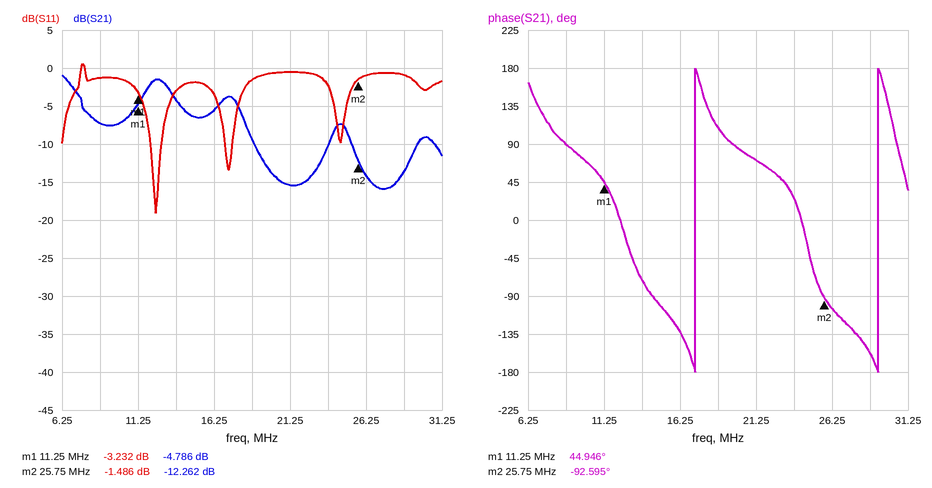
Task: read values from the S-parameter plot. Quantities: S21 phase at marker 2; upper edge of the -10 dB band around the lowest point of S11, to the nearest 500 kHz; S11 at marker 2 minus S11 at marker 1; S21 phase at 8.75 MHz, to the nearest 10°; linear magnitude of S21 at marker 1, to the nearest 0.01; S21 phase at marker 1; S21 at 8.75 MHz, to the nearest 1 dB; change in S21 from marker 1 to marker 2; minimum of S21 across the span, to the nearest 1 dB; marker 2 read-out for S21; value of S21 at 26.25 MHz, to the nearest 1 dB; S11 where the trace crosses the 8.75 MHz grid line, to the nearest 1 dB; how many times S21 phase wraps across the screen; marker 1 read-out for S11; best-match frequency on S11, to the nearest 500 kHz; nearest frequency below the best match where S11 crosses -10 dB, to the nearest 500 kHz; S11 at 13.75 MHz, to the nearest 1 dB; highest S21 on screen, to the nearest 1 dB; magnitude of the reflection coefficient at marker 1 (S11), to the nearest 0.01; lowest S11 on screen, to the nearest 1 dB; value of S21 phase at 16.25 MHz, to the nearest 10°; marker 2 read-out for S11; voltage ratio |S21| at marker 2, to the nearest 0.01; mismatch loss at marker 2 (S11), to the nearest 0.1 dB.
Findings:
-92.595°
13.0 MHz
1.746 dB
90°
0.58
44.946°
-7 dB
-7.476 dB
-16 dB
-12.262 dB
-14 dB
-1 dB
2
-3.232 dB
12.5 MHz
12.0 MHz
-3 dB
-1 dB
0.69
-19 dB
-130°
-1.486 dB
0.24
5.4 dB
